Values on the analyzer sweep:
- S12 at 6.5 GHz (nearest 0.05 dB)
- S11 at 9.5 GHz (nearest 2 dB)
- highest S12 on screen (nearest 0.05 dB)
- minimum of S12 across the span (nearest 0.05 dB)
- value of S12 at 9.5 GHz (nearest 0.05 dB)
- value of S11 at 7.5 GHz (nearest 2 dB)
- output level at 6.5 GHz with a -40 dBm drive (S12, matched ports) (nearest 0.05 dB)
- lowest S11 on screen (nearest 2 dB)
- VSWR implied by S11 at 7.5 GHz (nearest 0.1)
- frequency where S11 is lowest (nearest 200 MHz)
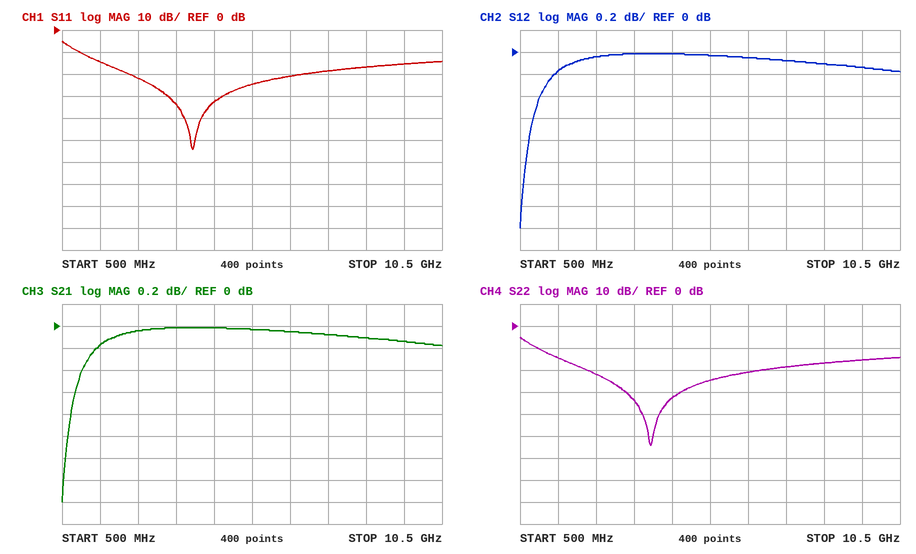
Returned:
-0.05 dB
-16 dB
0.00 dB
-1.60 dB
-0.15 dB
-18 dB
-40.05 dBm
-54 dB
1.3
4.0 GHz
